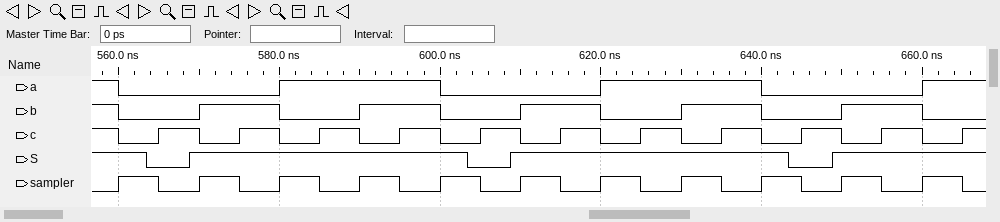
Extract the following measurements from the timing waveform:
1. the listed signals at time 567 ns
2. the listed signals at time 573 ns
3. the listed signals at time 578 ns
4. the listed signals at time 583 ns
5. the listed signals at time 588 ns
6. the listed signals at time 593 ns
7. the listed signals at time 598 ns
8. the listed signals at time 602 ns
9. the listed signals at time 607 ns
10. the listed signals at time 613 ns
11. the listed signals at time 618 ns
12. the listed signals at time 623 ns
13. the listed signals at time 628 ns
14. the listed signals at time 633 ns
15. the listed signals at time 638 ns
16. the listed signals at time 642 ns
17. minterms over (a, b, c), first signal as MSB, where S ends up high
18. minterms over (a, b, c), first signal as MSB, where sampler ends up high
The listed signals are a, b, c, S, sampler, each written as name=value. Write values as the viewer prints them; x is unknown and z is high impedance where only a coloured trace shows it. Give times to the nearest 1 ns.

a=0, b=0, c=1, S=0, sampler=0
a=0, b=1, c=0, S=1, sampler=1
a=0, b=1, c=1, S=1, sampler=0
a=1, b=0, c=0, S=1, sampler=1
a=1, b=0, c=1, S=1, sampler=0
a=1, b=1, c=0, S=1, sampler=1
a=1, b=1, c=1, S=1, sampler=0
a=0, b=0, c=0, S=1, sampler=1
a=0, b=0, c=1, S=0, sampler=0
a=0, b=1, c=0, S=1, sampler=1
a=0, b=1, c=1, S=1, sampler=0
a=1, b=0, c=0, S=1, sampler=1
a=1, b=0, c=1, S=1, sampler=0
a=1, b=1, c=0, S=1, sampler=1
a=1, b=1, c=1, S=1, sampler=0
a=0, b=0, c=0, S=1, sampler=1
1, 2, 3, 4, 5, 6, 7
0, 2, 4, 6
